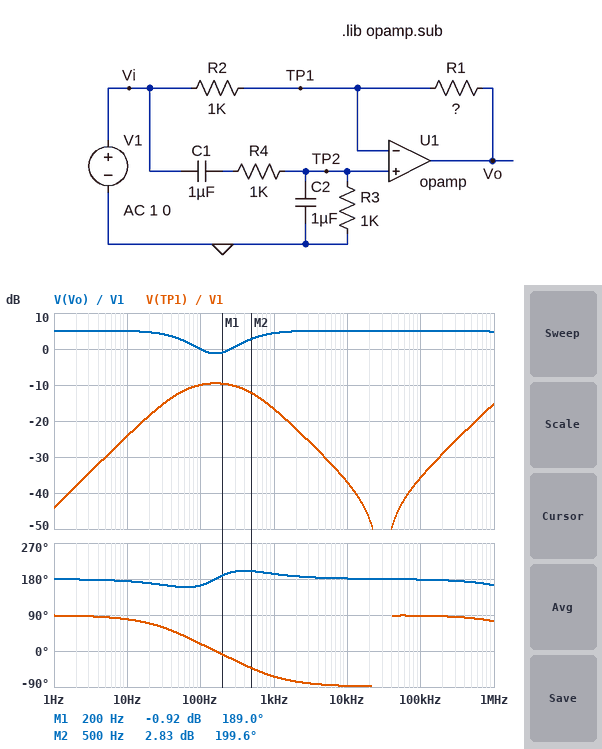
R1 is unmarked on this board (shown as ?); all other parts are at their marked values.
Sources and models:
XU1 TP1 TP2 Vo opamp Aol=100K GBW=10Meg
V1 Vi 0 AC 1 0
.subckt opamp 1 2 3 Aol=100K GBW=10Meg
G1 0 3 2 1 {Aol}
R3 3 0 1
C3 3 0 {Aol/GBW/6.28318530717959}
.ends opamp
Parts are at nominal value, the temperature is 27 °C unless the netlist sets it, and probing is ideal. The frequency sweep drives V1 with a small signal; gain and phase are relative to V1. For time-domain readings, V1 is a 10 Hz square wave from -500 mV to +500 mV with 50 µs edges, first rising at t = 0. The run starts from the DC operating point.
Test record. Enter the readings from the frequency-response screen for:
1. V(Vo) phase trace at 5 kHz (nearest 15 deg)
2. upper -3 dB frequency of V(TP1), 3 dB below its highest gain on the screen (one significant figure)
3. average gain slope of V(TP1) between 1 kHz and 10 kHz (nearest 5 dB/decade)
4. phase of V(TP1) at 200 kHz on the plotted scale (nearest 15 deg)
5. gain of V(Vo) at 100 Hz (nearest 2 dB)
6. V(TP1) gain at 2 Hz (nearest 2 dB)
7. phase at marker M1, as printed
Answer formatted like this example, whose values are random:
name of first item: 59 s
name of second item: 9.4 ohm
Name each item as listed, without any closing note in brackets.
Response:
V(Vo) phase trace at 5 kHz: 180 deg
upper -3 dB frequency of V(TP1), 3 dB below its highest gain on the screen: 500 Hz
average gain slope of V(TP1) between 1 kHz and 10 kHz: -20 dB/decade
phase of V(TP1) at 200 kHz on the plotted scale: 90 deg
gain of V(Vo) at 100 Hz: 0 dB
V(TP1) gain at 2 Hz: -38 dB
phase at marker M1, as printed: 189.0 deg
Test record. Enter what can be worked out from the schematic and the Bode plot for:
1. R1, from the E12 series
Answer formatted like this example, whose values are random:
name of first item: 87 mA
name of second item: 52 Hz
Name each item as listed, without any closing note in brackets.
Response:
R1, from the E12 series: 1.8 kΩ
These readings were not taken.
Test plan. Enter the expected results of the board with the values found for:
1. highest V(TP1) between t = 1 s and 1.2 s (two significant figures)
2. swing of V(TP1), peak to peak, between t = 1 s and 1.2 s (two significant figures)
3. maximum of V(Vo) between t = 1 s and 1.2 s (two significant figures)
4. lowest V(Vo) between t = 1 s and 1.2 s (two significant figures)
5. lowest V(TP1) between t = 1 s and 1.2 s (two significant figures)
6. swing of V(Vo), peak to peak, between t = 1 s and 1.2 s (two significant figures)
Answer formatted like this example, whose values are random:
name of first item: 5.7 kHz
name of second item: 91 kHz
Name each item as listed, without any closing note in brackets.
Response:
highest V(TP1) between t = 1 s and 1.2 s: 280 mV
swing of V(TP1), peak to peak, between t = 1 s and 1.2 s: 550 mV
maximum of V(Vo) between t = 1 s and 1.2 s: 900 mV
lowest V(Vo) between t = 1 s and 1.2 s: -900 mV
lowest V(TP1) between t = 1 s and 1.2 s: -280 mV
swing of V(Vo), peak to peak, between t = 1 s and 1.2 s: 1.8 V
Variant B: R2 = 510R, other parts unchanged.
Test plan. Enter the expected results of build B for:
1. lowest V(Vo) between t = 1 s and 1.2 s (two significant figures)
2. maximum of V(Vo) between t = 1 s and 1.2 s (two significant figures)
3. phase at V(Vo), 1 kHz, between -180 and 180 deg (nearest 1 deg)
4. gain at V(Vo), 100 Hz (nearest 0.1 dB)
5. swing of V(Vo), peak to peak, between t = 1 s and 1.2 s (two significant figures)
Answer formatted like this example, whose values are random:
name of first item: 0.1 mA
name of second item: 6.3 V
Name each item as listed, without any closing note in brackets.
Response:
lowest V(Vo) between t = 1 s and 1.2 s: -1.8 V
maximum of V(Vo) between t = 1 s and 1.2 s: 1.8 V
phase at V(Vo), 1 kHz, between -180 and 180 deg: -170 deg
gain at V(Vo), 100 Hz: 6.9 dB
swing of V(Vo), peak to peak, between t = 1 s and 1.2 s: 3.5 V
